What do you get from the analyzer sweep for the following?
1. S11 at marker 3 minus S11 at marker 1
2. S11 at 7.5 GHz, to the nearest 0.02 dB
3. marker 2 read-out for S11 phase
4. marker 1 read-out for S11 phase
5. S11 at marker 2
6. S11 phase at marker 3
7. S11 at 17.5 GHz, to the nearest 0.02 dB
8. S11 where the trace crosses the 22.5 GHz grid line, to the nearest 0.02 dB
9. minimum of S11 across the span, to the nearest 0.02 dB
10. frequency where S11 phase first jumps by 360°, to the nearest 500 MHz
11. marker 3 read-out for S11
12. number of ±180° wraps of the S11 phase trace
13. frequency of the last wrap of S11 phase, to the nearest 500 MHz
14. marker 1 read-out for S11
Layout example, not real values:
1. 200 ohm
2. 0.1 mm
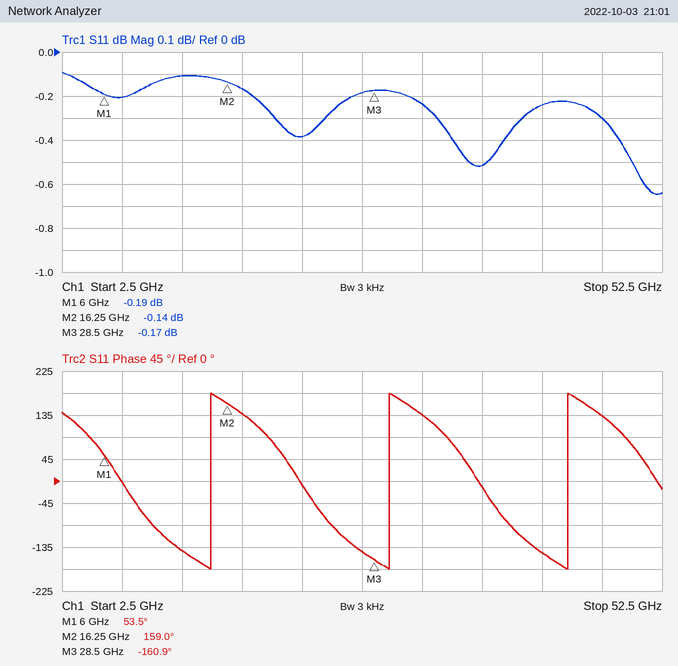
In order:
1. 0.02 dB
2. -0.20 dB
3. 159.0°
4. 53.5°
5. -0.14 dB
6. -160.9°
7. -0.16 dB
8. -0.38 dB
9. -0.64 dB
10. 15.0 GHz
11. -0.17 dB
12. 3
13. 44.5 GHz
14. -0.19 dB
